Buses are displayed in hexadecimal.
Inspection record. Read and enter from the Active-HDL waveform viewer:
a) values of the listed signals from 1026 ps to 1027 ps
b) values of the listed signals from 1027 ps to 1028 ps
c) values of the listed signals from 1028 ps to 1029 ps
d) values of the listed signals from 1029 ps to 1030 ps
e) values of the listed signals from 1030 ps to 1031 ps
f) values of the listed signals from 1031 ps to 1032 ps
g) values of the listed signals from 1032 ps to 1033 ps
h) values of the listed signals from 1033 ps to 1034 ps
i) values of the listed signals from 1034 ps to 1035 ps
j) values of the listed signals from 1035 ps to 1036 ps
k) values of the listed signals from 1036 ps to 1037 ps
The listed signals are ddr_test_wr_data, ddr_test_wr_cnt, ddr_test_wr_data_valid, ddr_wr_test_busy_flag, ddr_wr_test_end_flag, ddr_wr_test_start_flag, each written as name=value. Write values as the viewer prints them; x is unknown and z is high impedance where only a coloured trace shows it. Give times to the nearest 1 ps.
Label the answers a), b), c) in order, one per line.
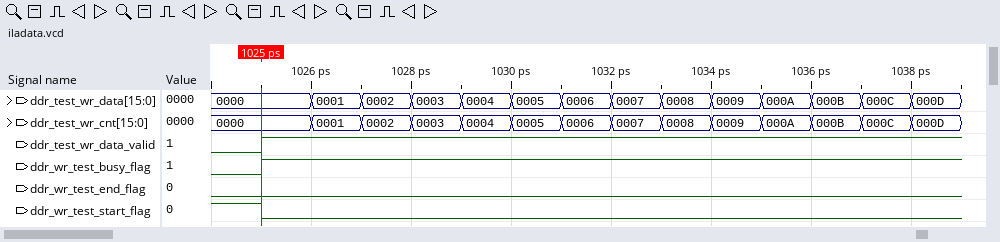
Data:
a) ddr_test_wr_data=0001, ddr_test_wr_cnt=0001, ddr_test_wr_data_valid=1, ddr_wr_test_busy_flag=1, ddr_wr_test_end_flag=0, ddr_wr_test_start_flag=0
b) ddr_test_wr_data=0002, ddr_test_wr_cnt=0002, ddr_test_wr_data_valid=1, ddr_wr_test_busy_flag=1, ddr_wr_test_end_flag=0, ddr_wr_test_start_flag=0
c) ddr_test_wr_data=0003, ddr_test_wr_cnt=0003, ddr_test_wr_data_valid=1, ddr_wr_test_busy_flag=1, ddr_wr_test_end_flag=0, ddr_wr_test_start_flag=0
d) ddr_test_wr_data=0004, ddr_test_wr_cnt=0004, ddr_test_wr_data_valid=1, ddr_wr_test_busy_flag=1, ddr_wr_test_end_flag=0, ddr_wr_test_start_flag=0
e) ddr_test_wr_data=0005, ddr_test_wr_cnt=0005, ddr_test_wr_data_valid=1, ddr_wr_test_busy_flag=1, ddr_wr_test_end_flag=0, ddr_wr_test_start_flag=0
f) ddr_test_wr_data=0006, ddr_test_wr_cnt=0006, ddr_test_wr_data_valid=1, ddr_wr_test_busy_flag=1, ddr_wr_test_end_flag=0, ddr_wr_test_start_flag=0
g) ddr_test_wr_data=0007, ddr_test_wr_cnt=0007, ddr_test_wr_data_valid=1, ddr_wr_test_busy_flag=1, ddr_wr_test_end_flag=0, ddr_wr_test_start_flag=0
h) ddr_test_wr_data=0008, ddr_test_wr_cnt=0008, ddr_test_wr_data_valid=1, ddr_wr_test_busy_flag=1, ddr_wr_test_end_flag=0, ddr_wr_test_start_flag=0
i) ddr_test_wr_data=0009, ddr_test_wr_cnt=0009, ddr_test_wr_data_valid=1, ddr_wr_test_busy_flag=1, ddr_wr_test_end_flag=0, ddr_wr_test_start_flag=0
j) ddr_test_wr_data=000A, ddr_test_wr_cnt=000A, ddr_test_wr_data_valid=1, ddr_wr_test_busy_flag=1, ddr_wr_test_end_flag=0, ddr_wr_test_start_flag=0
k) ddr_test_wr_data=000B, ddr_test_wr_cnt=000B, ddr_test_wr_data_valid=1, ddr_wr_test_busy_flag=1, ddr_wr_test_end_flag=0, ddr_wr_test_start_flag=0
